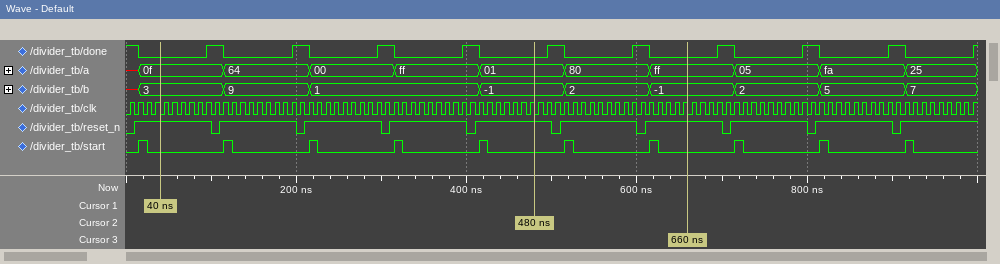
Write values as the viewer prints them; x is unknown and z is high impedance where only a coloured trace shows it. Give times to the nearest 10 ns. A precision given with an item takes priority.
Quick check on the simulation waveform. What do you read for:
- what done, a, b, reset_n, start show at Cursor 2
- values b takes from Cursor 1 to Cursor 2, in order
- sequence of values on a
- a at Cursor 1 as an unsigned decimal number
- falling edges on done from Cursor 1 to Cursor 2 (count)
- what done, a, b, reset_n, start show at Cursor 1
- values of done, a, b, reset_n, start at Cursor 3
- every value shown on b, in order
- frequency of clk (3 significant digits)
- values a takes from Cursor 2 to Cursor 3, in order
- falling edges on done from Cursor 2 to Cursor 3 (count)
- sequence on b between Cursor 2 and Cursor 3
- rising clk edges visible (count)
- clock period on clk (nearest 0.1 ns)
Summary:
done=0, a=01, b=-1, reset_n=1, start=0
3, 9, 1, -1
x, 0f, 64, 00, ff, 01, 80, ff, 05, fa, 25
15
4
done=0, a=0f, b=3, reset_n=1, start=0
done=0, a=ff, b=-1, reset_n=1, start=0
x, 3, 9, 1, -1, 2, -1, 2, 5, 7
100 MHz
01, 80, ff
2
-1, 2, -1
100
10 ns
